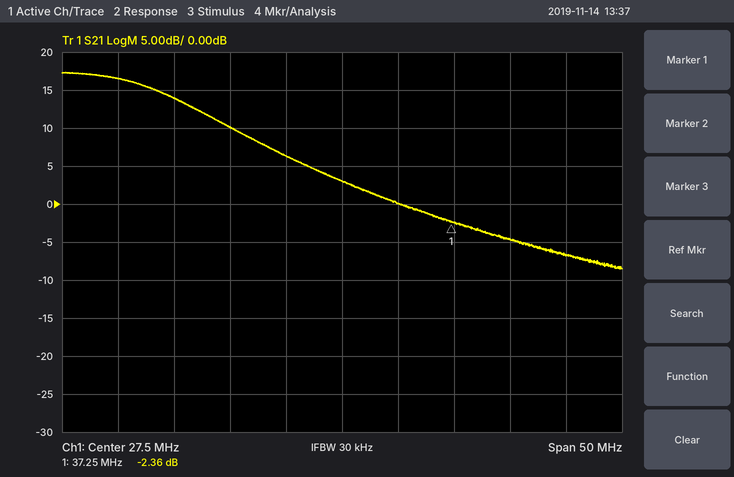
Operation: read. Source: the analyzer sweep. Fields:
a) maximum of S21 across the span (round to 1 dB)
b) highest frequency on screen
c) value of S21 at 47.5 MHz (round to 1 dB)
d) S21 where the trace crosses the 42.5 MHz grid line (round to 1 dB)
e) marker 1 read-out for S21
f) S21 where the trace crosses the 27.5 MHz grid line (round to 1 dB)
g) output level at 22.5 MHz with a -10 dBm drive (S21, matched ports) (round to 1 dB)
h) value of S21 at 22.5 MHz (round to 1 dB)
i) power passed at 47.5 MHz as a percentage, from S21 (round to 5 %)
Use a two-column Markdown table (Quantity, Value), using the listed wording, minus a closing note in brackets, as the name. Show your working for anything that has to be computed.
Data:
| Quantity | Value |
|---|---|
| maximum of S21 across the span | 17 dB |
| highest frequency on screen | 52.5 MHz |
| value of S21 at 47.5 MHz | -7 dB |
| S21 where the trace crosses the 42.5 MHz grid line | -5 dB |
| marker 1 read-out for S21 | -2.36 dB |
| S21 where the trace crosses the 27.5 MHz grid line | 3 dB |
| output level at 22.5 MHz with a -10 dBm drive (S21, matched ports) | -10 dBm + (6 dB) = -4 dBm |
| value of S21 at 22.5 MHz | 6 dB |
| power passed at 47.5 MHz as a percentage, from S21 | 10^(-7/10) ≈ 20 % |
